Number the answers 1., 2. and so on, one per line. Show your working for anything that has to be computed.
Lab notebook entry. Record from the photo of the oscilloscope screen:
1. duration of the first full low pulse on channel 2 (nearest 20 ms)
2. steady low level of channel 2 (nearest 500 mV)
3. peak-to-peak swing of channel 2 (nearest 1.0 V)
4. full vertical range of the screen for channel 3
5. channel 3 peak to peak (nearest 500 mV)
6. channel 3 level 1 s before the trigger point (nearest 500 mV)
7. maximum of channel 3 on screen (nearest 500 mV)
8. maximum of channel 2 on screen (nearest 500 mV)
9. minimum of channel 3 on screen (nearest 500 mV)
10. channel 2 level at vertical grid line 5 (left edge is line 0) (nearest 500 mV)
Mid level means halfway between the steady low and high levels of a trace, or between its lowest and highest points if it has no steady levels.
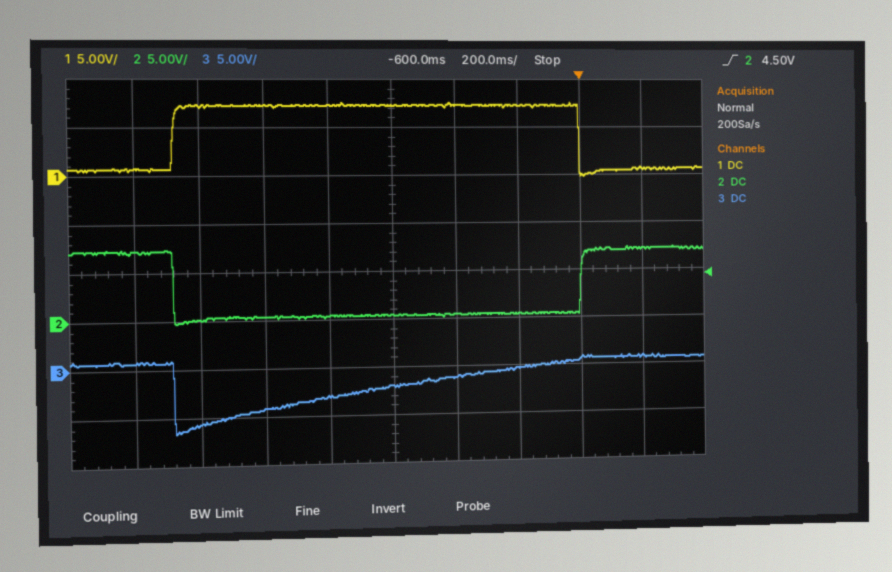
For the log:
1. 1.28 s
2. 500 mV
3. 8.0 V
4. 40 V
5. 1.0 V − (-6.5 V) = 7.5 V
6. -4.0 V
7. 1.0 V
8. 7.5 V
9. -6.5 V
10. 500 mV
